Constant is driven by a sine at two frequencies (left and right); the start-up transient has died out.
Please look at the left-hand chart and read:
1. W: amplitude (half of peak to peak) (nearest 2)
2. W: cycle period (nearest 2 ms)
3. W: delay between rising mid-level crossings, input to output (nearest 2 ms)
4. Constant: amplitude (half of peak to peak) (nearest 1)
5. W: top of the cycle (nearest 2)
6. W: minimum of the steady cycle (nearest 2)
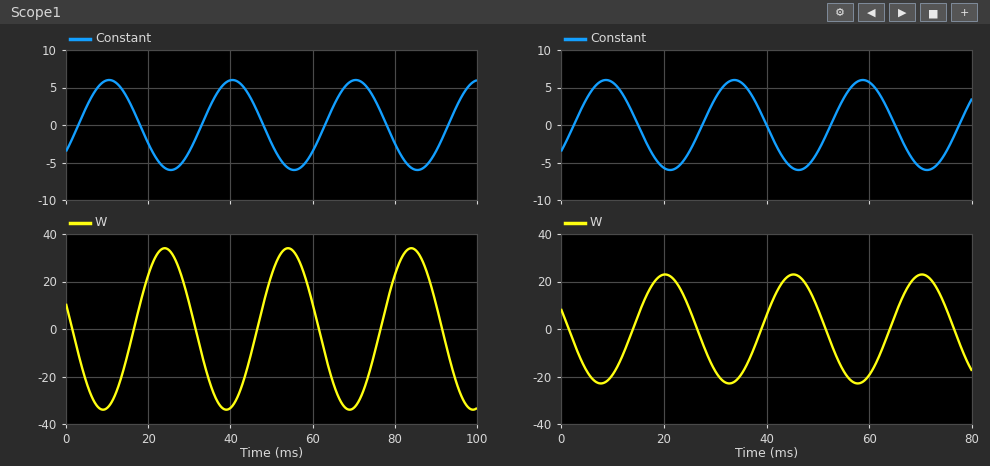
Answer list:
34
30 ms
14 ms
6
34
-34
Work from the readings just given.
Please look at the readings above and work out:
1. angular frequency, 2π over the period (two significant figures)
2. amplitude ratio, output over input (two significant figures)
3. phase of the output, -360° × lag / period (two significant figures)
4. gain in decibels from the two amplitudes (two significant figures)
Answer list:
0.21 rad/ms
5.7
-170°
15 dB
